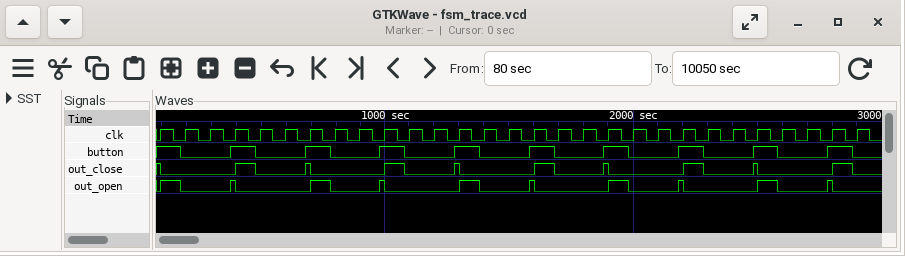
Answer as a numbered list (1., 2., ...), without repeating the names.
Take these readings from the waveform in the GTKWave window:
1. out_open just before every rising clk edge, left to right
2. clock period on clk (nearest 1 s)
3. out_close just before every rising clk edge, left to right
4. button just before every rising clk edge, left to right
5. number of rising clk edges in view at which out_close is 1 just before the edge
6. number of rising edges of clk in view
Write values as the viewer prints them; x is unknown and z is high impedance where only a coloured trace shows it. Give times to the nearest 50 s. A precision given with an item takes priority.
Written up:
1. 0 0 0 1 0 0 0 0 0 1 0 0 0 0 0 1 0 0 0 0 0 1 0 0 0 0 0 1 0
2. 100 s
3. 1 0 0 0 0 0 1 0 0 0 0 0 1 0 0 0 0 0 1 0 0 0 0 0 1 0 0 0 0
4. 1 0 0 1 0 0 1 0 0 1 0 0 1 0 0 1 0 0 1 0 0 1 0 0 1 0 0 1 0
5. 5
6. 29
